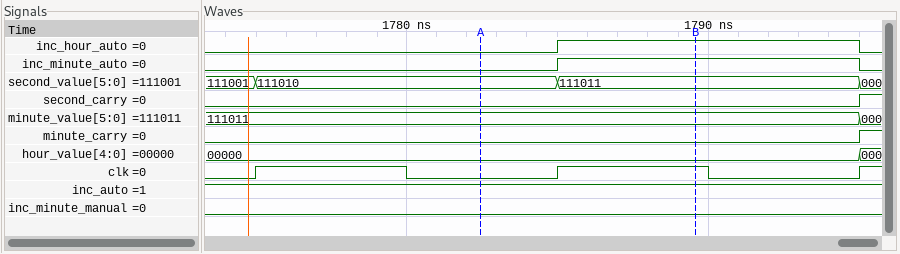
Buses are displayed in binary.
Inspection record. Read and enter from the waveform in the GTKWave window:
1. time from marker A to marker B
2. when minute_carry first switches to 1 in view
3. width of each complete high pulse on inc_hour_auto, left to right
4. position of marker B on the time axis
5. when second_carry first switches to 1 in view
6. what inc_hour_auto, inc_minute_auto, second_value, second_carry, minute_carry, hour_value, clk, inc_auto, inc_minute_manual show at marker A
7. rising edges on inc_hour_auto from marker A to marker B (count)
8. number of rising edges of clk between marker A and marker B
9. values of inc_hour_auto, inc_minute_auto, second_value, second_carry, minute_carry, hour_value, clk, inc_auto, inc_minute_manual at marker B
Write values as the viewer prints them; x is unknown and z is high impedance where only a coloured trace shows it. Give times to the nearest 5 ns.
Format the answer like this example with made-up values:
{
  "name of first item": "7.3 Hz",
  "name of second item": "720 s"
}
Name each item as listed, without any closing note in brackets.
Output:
{
  "time from marker A to marker B": "5 ns",
  "when minute_carry first switches to 1 in view": "1795 ns",
  "width of each complete high pulse on inc_hour_auto, left to right": "10 ns",
  "position of marker B on the time axis": "1790 ns",
  "when second_carry first switches to 1 in view": "1795 ns",
  "what inc_hour_auto, inc_minute_auto, second_value, second_carry, minute_carry, hour_value, clk, inc_auto, inc_minute_manual show at marker A": "inc_hour_auto=0, inc_minute_auto=0, second_value=111010, second_carry=0, minute_carry=0, hour_value=00000, clk=0, inc_auto=1, inc_minute_manual=0",
  "rising edges on inc_hour_auto from marker A to marker B": "1",
  "number of rising edges of clk between marker A and marker B": "1",
  "values of inc_hour_auto, inc_minute_auto, second_value, second_carry, minute_carry, hour_value, clk, inc_auto, inc_minute_manual at marker B": "inc_hour_auto=1, inc_minute_auto=1, second_value=111011, second_carry=0, minute_carry=0, hour_value=00000, clk=1, inc_auto=1, inc_minute_manual=0"
}
